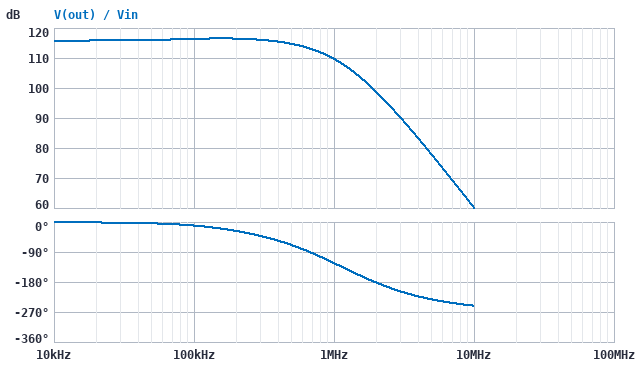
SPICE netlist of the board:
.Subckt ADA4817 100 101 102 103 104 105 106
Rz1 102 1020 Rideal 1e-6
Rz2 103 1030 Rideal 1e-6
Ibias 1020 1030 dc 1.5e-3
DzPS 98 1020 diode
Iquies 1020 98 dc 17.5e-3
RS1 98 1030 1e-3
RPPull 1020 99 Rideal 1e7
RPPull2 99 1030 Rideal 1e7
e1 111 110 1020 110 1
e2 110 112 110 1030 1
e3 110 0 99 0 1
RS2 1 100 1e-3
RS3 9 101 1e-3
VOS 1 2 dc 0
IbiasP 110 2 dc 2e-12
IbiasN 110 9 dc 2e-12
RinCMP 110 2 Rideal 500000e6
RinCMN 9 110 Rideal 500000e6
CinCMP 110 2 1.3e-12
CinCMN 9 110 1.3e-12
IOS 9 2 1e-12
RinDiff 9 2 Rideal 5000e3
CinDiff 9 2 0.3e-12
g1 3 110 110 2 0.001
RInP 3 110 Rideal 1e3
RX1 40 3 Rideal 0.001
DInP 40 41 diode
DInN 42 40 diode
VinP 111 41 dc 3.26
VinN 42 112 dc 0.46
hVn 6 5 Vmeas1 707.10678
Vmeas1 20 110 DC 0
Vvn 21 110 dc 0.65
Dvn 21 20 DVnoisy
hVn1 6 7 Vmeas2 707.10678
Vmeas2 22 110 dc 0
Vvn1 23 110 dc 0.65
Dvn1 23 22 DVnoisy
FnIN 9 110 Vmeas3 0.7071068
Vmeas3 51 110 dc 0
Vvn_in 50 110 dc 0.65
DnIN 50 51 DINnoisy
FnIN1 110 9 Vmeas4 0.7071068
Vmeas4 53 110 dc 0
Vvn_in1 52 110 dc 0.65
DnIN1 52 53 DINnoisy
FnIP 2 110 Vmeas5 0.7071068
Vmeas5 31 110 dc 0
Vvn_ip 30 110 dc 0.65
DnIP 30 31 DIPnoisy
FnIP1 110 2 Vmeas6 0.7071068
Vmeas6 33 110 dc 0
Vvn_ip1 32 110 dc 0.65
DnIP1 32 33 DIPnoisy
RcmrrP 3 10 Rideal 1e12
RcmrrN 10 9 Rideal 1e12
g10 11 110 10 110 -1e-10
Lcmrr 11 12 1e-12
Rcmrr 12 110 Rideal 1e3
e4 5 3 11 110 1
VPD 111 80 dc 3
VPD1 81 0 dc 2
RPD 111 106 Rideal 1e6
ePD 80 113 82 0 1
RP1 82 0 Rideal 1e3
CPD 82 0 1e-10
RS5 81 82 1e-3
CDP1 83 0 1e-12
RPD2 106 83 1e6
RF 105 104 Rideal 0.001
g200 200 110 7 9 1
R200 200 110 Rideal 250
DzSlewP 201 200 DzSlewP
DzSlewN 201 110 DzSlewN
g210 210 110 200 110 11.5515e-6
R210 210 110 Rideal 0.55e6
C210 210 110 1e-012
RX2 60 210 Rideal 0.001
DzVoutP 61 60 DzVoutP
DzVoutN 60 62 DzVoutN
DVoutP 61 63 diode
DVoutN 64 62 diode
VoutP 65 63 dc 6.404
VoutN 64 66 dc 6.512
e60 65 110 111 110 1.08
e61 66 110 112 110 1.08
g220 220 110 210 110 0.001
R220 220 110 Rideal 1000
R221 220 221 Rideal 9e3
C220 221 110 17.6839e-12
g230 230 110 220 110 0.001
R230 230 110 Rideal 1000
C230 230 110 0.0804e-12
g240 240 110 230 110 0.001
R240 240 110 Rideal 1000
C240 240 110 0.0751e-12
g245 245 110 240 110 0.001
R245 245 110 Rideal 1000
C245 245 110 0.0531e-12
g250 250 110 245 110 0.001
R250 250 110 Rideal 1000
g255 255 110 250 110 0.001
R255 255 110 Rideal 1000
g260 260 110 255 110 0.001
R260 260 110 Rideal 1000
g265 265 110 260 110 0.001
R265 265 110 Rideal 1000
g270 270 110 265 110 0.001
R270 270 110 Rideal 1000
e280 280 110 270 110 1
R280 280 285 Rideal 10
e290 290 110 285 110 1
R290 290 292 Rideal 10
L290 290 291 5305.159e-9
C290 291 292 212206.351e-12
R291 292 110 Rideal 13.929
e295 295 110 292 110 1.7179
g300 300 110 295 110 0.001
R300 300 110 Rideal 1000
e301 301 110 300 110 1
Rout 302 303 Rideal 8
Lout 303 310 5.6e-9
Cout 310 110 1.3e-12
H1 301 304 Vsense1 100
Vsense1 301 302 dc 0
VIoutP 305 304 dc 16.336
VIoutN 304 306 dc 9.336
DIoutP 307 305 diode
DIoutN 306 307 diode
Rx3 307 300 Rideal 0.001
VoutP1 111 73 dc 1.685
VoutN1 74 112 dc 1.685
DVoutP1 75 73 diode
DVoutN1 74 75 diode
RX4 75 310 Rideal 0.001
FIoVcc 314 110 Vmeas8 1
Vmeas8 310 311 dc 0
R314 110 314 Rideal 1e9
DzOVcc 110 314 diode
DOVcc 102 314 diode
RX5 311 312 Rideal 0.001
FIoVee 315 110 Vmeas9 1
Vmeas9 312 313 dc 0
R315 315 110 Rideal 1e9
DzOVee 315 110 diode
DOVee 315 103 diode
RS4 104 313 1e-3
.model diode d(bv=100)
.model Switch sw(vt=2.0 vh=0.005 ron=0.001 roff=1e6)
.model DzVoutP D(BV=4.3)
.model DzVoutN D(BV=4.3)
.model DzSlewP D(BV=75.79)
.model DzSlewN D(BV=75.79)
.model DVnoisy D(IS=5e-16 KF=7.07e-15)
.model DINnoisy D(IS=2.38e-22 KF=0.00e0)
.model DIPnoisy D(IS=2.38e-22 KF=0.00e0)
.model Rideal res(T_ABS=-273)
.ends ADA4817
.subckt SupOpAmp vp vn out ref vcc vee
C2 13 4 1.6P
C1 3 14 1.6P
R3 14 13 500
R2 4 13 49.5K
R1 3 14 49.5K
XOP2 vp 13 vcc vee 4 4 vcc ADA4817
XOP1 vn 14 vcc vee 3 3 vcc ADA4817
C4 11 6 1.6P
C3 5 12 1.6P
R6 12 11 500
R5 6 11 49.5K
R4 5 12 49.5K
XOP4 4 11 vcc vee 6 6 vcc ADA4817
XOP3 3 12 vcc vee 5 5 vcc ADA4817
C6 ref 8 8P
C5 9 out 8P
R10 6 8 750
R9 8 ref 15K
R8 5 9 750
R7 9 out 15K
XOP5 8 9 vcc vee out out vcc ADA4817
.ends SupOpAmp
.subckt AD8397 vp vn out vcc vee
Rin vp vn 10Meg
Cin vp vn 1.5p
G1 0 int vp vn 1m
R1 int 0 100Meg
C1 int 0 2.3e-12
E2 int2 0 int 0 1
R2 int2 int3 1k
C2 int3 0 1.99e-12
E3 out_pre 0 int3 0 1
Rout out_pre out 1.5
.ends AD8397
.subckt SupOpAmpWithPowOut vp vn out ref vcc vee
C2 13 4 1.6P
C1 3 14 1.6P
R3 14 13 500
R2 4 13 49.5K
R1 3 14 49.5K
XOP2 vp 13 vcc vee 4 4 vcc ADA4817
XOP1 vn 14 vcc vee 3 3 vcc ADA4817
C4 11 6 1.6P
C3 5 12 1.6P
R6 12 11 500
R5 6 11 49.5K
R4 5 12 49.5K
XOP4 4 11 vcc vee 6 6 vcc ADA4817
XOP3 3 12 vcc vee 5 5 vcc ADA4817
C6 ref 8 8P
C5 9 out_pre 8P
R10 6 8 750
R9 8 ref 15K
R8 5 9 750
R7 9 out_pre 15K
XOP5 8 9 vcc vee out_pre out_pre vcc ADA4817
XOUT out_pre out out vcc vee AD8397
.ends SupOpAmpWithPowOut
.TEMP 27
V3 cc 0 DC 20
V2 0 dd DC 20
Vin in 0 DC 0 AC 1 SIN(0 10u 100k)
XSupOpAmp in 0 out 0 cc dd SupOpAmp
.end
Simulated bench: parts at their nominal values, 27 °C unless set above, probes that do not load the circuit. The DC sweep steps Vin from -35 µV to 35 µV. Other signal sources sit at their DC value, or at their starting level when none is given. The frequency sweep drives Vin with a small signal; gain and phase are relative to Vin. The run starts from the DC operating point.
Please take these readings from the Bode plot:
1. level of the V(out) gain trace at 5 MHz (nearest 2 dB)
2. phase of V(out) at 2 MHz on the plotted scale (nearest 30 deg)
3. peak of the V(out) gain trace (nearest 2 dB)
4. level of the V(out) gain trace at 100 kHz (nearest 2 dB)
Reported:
78 dB
-180 deg
116 dB
116 dB
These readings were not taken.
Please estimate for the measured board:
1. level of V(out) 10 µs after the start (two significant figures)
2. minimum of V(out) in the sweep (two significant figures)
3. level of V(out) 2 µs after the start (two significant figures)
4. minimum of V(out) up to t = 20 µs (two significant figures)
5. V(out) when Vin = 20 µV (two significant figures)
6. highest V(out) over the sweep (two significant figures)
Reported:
-1.2 V
-19 V
5.6 V
-6.6 V
12 V
19 V
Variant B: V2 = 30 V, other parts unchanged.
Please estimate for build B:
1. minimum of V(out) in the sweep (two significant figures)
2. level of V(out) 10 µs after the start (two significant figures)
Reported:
-22 V
-1.3 V
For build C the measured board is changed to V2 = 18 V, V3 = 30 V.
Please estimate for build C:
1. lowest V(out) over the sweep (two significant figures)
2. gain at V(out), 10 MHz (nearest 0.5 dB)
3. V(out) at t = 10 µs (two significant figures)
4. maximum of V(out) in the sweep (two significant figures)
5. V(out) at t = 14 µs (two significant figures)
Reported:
-17 V
60.0 dB
-1.1 V
22 V
4.9 V
